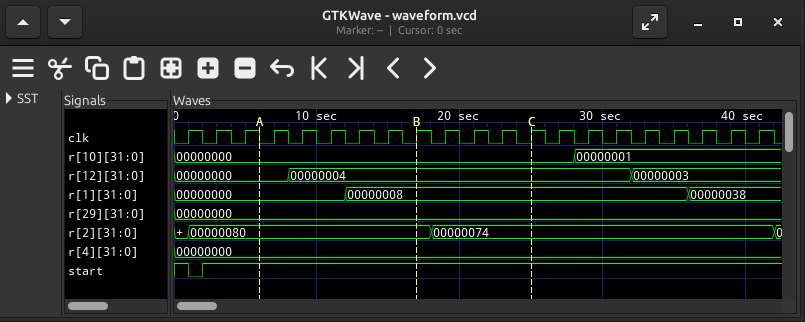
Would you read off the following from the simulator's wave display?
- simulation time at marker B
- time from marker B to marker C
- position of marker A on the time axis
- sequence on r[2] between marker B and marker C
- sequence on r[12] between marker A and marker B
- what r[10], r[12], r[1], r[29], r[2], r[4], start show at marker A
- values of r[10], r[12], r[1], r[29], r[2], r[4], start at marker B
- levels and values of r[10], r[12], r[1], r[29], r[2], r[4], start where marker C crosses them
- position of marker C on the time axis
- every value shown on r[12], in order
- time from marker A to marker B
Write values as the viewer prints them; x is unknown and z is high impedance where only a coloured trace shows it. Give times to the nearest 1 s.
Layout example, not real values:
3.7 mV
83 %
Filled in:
17 s
8 s
6 s
00000080, 00000074
00000000, 00000004
r[10]=00000000, r[12]=00000000, r[1]=00000000, r[29]=00000000, r[2]=00000080, r[4]=00000000, start=1
r[10]=00000000, r[12]=00000004, r[1]=00000008, r[29]=00000000, r[2]=00000080, r[4]=00000000, start=1
r[10]=00000000, r[12]=00000004, r[1]=00000008, r[29]=00000000, r[2]=00000074, r[4]=00000000, start=1
25 s
00000000, 00000004, 00000003
11 s
